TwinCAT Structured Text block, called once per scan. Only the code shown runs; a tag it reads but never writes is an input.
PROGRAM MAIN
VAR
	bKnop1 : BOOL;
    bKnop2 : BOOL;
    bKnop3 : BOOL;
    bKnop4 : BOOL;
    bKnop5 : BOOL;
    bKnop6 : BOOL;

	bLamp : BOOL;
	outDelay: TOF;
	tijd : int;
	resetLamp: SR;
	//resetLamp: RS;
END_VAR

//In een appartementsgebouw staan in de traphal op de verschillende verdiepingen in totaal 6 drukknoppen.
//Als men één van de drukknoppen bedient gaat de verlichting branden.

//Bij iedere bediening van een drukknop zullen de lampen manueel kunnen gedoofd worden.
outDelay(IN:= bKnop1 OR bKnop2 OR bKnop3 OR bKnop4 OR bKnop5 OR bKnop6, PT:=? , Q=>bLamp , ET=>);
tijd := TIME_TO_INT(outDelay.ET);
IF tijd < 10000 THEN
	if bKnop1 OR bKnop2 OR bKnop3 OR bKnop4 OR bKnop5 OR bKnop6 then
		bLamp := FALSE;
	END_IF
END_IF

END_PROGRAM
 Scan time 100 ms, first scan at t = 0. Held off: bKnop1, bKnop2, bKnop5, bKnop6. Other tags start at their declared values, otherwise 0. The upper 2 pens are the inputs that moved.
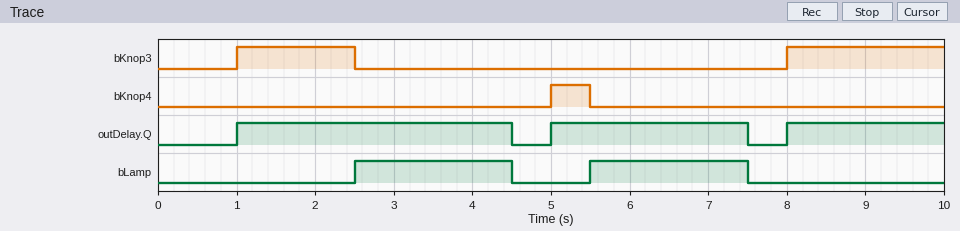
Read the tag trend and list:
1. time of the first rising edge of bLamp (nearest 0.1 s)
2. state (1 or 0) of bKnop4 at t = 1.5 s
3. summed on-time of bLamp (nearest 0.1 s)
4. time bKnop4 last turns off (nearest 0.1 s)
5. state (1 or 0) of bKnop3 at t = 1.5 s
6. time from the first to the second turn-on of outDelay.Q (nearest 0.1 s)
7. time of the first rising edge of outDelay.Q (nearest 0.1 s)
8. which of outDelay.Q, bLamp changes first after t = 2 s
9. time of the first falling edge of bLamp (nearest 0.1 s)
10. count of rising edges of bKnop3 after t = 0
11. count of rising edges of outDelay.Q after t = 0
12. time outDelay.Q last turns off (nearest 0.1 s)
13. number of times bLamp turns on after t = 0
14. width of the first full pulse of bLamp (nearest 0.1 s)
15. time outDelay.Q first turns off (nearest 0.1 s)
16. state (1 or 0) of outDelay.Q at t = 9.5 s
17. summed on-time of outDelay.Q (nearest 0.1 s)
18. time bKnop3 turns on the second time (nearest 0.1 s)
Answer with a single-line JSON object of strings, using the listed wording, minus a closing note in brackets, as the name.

{"time of the first rising edge of bLamp": "2.5 s", "state (1 or 0) of bKnop4 at t = 1.5 s": "0", "summed on-time of bLamp": "4.0 s", "time bKnop4 last turns off": "5.5 s", "state (1 or 0) of bKnop3 at t = 1.5 s": "1", "time from the first to the second turn-on of outDelay.Q": "4.0 s", "time of the first rising edge of outDelay.Q": "1.0 s", "which of outDelay.Q, bLamp changes first after t = 2 s": "bLamp", "time of the first falling edge of bLamp": "4.5 s", "count of rising edges of bKnop3 after t = 0": "2", "count of rising edges of outDelay.Q after t = 0": "3", "time outDelay.Q last turns off": "7.5 s", "number of times bLamp turns on after t = 0": "2", "width of the first full pulse of bLamp": "2.0 s", "time outDelay.Q first turns off": "4.5 s", "state (1 or 0) of outDelay.Q at t = 9.5 s": "1", "summed on-time of outDelay.Q": "8.0 s", "time bKnop3 turns on the second time": "8.0 s"}
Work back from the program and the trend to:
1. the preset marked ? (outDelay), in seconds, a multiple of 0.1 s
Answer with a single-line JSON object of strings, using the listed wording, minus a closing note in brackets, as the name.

{"the preset marked ? (outDelay), in seconds, a multiple of 0.1 s": "2.0 s"}
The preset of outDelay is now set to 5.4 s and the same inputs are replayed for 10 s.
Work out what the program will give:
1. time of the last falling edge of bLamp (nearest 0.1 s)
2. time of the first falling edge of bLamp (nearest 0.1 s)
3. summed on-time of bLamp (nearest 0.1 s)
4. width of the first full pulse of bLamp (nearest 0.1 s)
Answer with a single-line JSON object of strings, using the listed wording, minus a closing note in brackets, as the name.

{"time of the last falling edge of bLamp": "8.0 s", "time of the first falling edge of bLamp": "5.0 s", "summed on-time of bLamp": "5.0 s", "width of the first full pulse of bLamp": "2.5 s"}
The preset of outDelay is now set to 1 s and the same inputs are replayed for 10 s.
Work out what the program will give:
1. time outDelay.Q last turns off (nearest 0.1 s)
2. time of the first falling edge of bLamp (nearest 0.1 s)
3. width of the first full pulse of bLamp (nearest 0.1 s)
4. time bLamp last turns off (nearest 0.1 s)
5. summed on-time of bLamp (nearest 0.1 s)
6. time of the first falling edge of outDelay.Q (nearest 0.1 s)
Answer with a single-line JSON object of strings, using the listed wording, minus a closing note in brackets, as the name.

{"time outDelay.Q last turns off": "6.5 s", "time of the first falling edge of bLamp": "3.5 s", "width of the first full pulse of bLamp": "1.0 s", "time bLamp last turns off": "6.5 s", "summed on-time of bLamp": "2.0 s", "time of the first falling edge of outDelay.Q": "3.5 s"}
